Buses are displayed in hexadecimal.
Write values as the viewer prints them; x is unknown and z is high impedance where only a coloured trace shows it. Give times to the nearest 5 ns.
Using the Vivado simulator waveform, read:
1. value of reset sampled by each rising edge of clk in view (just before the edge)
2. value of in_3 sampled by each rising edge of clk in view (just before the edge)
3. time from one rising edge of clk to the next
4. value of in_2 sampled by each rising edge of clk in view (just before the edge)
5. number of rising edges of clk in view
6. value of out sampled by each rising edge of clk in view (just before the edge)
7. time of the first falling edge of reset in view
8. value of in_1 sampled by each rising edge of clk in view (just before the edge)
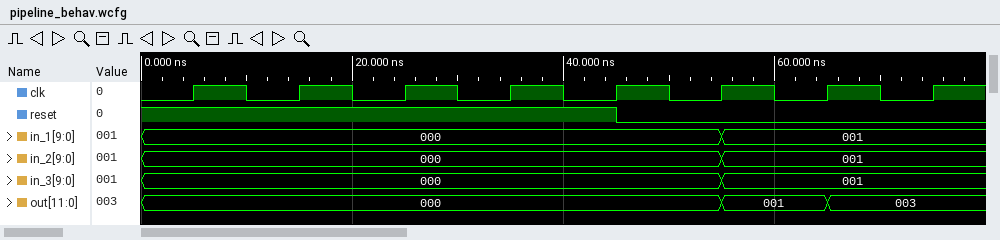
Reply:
1 1 1 1 1 0 0 0
000, 000, 000, 000, 000, 000, 001, 001
10 ns
000, 000, 000, 000, 000, 000, 001, 001
8
000, 000, 000, 000, 000, 000, 001, 003
45 ns
000, 000, 000, 000, 000, 000, 001, 001
